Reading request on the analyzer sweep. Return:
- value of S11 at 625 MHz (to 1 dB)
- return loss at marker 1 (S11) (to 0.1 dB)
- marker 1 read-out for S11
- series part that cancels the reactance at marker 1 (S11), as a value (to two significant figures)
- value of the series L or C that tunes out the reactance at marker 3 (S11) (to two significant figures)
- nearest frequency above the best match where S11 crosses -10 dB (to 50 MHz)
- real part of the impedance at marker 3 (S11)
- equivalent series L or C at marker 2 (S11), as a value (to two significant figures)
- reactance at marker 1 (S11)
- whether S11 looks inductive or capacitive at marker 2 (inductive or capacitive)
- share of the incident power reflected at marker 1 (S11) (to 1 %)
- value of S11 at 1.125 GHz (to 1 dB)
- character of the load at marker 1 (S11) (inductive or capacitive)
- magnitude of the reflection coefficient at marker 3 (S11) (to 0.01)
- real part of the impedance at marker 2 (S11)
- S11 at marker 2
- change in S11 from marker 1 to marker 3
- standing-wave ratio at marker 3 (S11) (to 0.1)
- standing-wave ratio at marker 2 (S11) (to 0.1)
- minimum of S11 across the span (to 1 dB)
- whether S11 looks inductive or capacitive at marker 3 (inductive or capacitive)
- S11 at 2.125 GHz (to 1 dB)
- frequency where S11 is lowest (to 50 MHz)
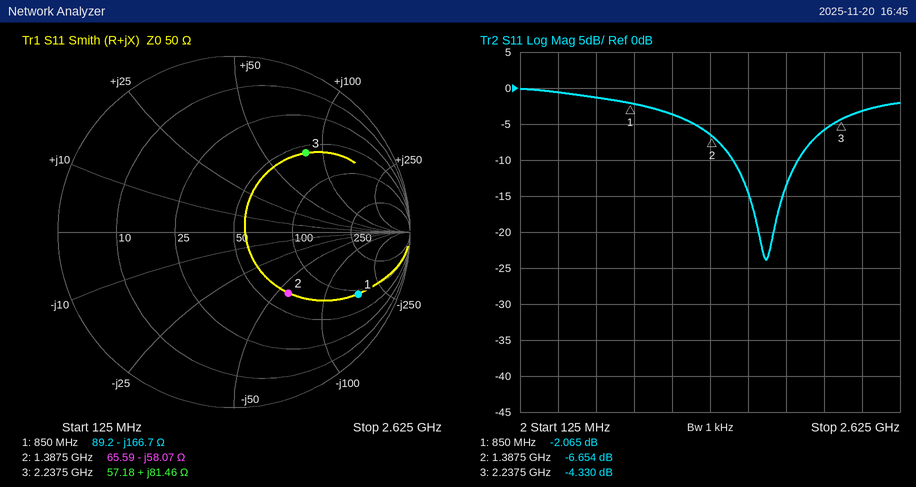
-1 dB
2.1 dB
-2.065 dB
31 nH
870 fF
1.95 GHz
57.18 Ω
2.0 pF
-166.7 Ω
capacitive
62 %
-4 dB
capacitive
0.61
65.59 Ω
-6.654 dB
-2.265 dB
4.1
2.7
-24 dB
inductive
-6 dB
1.75 GHz
